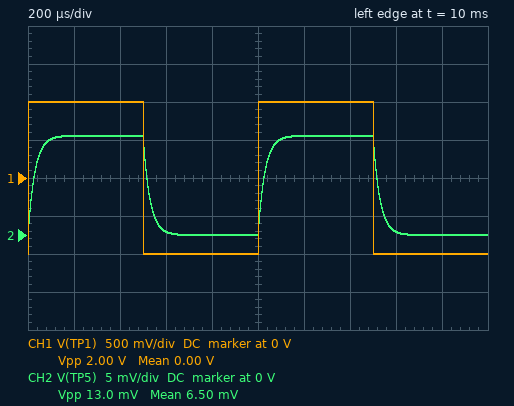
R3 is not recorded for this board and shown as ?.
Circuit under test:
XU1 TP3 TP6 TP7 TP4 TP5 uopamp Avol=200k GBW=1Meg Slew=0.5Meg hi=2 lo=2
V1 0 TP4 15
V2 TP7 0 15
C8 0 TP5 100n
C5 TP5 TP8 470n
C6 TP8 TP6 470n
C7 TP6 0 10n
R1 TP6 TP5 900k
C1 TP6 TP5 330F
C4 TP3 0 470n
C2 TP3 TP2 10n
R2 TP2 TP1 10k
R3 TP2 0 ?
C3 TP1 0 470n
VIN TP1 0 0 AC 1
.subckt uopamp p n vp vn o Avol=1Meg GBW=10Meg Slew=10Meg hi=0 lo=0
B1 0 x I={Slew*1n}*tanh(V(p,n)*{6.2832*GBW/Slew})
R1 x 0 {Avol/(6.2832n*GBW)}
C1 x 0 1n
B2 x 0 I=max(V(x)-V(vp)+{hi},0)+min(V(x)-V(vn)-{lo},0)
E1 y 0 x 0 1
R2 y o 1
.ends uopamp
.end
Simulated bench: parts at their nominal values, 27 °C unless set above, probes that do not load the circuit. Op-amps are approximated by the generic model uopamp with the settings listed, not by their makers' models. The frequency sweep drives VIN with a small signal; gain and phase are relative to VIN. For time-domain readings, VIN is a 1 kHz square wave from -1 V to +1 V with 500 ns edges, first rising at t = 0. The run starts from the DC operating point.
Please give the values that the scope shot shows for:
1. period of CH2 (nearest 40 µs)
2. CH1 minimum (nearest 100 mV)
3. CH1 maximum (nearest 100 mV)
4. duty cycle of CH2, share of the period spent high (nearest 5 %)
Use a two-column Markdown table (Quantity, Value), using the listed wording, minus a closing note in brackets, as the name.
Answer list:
| Quantity | Value |
|---|---|
| period of CH2 | 1.00 ms |
| CH1 minimum | -1.0 V |
| CH1 maximum | 1.0 V |
| duty cycle of CH2, share of the period spent high | 50 % |
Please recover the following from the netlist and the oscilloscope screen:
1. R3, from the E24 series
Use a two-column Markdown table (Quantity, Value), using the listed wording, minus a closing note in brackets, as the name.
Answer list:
| Quantity | Value |
|---|---|
| R3, from the E24 series | 4.3 kΩ |
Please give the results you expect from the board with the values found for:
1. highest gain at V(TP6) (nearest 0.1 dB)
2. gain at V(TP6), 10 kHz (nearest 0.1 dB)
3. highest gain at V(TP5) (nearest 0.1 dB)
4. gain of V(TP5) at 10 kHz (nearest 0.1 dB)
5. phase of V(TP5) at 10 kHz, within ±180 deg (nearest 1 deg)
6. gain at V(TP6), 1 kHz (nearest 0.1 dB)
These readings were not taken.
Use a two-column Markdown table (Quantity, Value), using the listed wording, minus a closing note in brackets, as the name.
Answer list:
| Quantity | Value |
|---|---|
| highest gain at V(TP6) | -44.1 dB |
| gain at V(TP6), 10 kHz | -50.5 dB |
| highest gain at V(TP5) | -43.7 dB |
| gain of V(TP5) at 10 kHz | -50.2 dB |
| phase of V(TP5) at 10 kHz, within ±180 deg | -62 deg |
| gain at V(TP6), 1 kHz | -44.2 dB |
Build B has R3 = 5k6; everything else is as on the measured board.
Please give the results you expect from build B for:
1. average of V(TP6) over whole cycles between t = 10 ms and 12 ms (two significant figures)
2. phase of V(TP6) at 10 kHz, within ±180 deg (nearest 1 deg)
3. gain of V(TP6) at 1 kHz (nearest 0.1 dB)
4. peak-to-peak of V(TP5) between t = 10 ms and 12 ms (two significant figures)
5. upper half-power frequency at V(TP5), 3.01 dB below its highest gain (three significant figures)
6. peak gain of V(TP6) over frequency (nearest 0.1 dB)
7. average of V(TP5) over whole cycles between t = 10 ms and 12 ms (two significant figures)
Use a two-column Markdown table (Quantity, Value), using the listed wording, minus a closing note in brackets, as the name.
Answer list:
| Quantity | Value |
|---|---|
| average of V(TP6) over whole cycles between t = 10 ms and 12 ms | 7.5 mV |
| phase of V(TP6) at 10 kHz, within ±180 deg | -66 deg |
| gain of V(TP6) at 1 kHz | -42.7 dB |
| peak-to-peak of V(TP5) between t = 10 ms and 12 ms | 16 mV |
| upper half-power frequency at V(TP5), 3.01 dB below its highest gain | 4.53 kHz |
| peak gain of V(TP6) over frequency | -42.5 dB |
| average of V(TP5) over whole cycles between t = 10 ms and 12 ms | 7.8 mV |
